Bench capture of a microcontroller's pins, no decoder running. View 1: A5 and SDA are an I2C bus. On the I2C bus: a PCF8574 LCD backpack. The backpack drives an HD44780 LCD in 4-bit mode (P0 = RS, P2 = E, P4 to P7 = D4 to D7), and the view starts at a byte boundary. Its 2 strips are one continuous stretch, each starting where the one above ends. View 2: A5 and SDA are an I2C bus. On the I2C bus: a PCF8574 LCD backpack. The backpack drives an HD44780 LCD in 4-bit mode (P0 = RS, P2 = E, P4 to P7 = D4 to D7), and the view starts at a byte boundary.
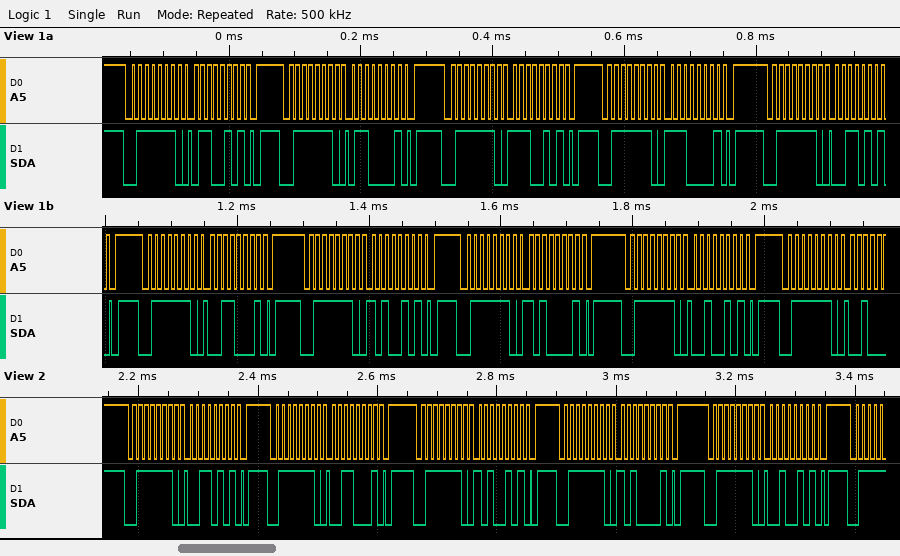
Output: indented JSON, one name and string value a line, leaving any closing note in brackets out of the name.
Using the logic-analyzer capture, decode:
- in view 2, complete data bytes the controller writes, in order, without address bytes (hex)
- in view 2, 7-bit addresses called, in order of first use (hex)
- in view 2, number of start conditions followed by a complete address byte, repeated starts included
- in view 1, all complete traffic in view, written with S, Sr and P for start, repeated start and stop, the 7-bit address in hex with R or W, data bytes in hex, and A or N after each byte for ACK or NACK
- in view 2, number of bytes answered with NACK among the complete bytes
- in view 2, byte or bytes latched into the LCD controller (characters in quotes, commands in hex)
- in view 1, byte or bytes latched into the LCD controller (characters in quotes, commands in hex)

{
  "in view 2, complete data bytes the controller writes, in order, without address bytes": "35 31 A5 A1 25",
  "in view 2, 7-bit addresses called, in order of first use": "0x3F",
  "in view 2, number of start conditions followed by a complete address byte, repeated starts included": "5",
  "in view 1, all complete traffic in view, written with S, Sr and P for start, repeated start and stop, the 7-bit address in hex with R or W, data bytes in hex, and A or N after each byte for ACK or NACK": "S 3FW A 65 A P S 3FW A 61 A P S 3FW A E5 A P S 3FW A E1 A P S 3FW A 35 A P S 3FW A 31 A P S 3FW A A5 A P S 3FW A A1 A P S 3FW A 25 A P S 3FW A",
  "in view 2, number of bytes answered with NACK among the complete bytes": "0",
  "in view 2, byte or bytes latched into the LCD controller": "':'",
  "in view 1, byte or bytes latched into the LCD controller": "'n' ':'"
}
